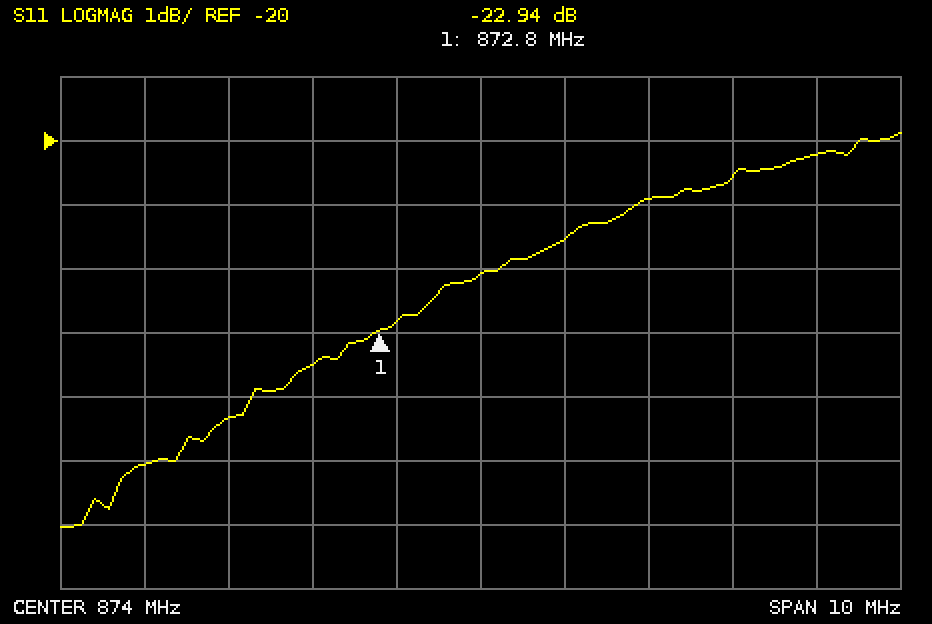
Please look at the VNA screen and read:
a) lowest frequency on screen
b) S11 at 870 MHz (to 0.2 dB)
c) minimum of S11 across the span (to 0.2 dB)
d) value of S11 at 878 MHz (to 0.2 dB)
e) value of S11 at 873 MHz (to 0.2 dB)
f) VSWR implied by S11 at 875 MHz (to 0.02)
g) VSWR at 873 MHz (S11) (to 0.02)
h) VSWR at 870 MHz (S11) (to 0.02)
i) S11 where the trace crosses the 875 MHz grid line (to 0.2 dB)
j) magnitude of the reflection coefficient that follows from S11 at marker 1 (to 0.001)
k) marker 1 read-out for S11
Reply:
869 MHz
-25.0 dB
-26.0 dB
-20.2 dB
-22.8 dB
1.18
1.16
1.12
-21.6 dB
0.071
-22.94 dB
